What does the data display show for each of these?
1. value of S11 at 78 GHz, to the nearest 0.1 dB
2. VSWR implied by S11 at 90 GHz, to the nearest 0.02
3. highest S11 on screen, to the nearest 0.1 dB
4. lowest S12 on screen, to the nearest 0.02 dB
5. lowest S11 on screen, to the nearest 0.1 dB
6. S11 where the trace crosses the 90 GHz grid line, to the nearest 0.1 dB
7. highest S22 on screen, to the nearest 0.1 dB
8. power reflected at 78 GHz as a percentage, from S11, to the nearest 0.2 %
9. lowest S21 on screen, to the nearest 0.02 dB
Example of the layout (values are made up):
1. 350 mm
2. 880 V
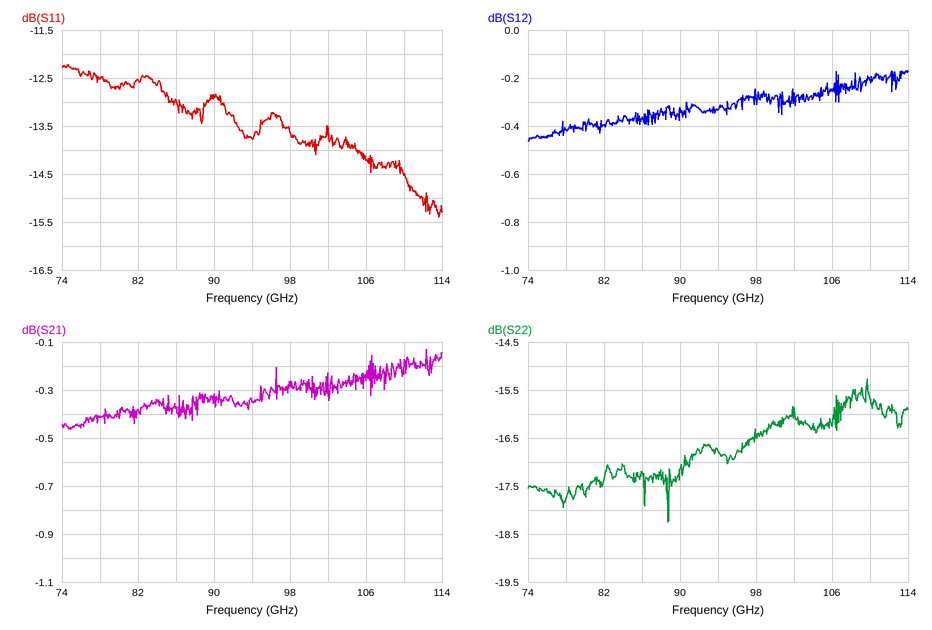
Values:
1. -12.5 dB
2. 1.58
3. -12.2 dB
4. -0.46 dB
5. -15.4 dB
6. -12.9 dB
7. -15.3 dB
8. 5.6 %
9. -0.46 dB
